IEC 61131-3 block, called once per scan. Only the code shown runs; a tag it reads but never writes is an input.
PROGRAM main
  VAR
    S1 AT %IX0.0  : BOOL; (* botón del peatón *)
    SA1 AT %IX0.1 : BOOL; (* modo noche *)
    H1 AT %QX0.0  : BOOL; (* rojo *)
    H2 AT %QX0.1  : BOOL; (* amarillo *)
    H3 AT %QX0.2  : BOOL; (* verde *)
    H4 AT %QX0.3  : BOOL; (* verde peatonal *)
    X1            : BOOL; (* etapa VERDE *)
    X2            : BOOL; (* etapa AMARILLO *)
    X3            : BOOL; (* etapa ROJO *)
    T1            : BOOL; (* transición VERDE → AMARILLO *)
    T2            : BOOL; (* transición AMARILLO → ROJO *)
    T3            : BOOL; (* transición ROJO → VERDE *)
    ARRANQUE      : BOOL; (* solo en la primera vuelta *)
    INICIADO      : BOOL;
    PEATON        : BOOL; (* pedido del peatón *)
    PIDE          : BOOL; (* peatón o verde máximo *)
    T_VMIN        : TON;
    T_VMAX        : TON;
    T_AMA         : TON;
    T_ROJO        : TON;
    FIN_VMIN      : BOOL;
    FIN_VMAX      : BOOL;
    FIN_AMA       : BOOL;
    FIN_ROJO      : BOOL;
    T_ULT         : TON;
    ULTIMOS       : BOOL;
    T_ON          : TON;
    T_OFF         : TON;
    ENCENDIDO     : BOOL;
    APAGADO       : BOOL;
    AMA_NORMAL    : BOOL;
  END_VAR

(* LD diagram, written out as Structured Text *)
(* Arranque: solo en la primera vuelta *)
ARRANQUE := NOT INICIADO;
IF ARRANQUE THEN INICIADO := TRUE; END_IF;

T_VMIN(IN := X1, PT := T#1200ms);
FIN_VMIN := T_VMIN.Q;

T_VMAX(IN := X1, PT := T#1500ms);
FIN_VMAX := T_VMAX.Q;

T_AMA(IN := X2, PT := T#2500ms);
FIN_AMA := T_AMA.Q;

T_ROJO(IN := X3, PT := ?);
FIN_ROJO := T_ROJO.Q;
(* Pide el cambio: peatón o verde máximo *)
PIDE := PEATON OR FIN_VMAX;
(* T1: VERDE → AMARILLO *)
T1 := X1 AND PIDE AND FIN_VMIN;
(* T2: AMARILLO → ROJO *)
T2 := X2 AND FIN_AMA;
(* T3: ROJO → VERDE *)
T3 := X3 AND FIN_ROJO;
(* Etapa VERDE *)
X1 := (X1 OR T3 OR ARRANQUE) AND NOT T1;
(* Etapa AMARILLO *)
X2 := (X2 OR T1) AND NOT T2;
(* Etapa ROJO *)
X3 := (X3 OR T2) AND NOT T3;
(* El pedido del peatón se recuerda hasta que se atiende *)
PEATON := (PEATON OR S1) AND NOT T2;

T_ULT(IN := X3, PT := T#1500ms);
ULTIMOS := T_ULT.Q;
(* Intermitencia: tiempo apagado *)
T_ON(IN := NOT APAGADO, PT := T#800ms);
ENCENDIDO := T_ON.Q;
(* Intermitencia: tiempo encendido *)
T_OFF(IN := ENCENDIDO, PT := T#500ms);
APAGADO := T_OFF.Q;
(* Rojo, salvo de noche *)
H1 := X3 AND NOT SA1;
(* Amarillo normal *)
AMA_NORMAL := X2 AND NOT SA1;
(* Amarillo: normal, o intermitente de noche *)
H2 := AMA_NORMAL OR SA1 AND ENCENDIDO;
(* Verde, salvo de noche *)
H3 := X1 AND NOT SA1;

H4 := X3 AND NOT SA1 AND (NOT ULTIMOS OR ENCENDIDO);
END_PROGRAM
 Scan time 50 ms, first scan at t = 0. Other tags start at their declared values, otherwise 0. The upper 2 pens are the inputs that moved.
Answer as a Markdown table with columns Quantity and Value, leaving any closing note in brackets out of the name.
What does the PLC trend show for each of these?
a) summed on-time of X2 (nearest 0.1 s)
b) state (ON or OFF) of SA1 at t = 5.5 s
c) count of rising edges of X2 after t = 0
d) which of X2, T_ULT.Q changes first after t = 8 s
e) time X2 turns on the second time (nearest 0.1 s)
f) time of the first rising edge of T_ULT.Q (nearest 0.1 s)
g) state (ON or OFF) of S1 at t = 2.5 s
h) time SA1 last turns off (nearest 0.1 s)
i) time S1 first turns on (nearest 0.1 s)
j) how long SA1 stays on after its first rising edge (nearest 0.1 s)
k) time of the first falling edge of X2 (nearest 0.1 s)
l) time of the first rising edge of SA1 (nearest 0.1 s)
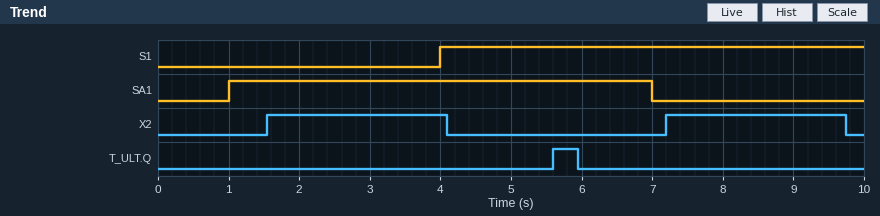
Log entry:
| Quantity | Value |
|---|---|
| summed on-time of X2 | 5.1 s |
| state (ON or OFF) of SA1 at t = 5.5 s | ON |
| count of rising edges of X2 after t = 0 | 2 |
| which of X2, T_ULT.Q changes first after t = 8 s | X2 |
| time X2 turns on the second time | 7.2 s |
| time of the first rising edge of T_ULT.Q | 5.6 s |
| state (ON or OFF) of S1 at t = 2.5 s | OFF |
| time SA1 last turns off | 7.0 s |
| time S1 first turns on | 4.0 s |
| how long SA1 stays on after its first rising edge | 6.0 s |
| time of the first falling edge of X2 | 4.1 s |
| time of the first rising edge of SA1 | 1.0 s |
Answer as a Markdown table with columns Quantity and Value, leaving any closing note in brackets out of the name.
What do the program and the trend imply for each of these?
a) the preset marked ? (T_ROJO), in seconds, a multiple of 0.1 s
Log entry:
| Quantity | Value |
|---|---|
| the preset marked ? (T_ROJO), in seconds, a multiple of 0.1 s | 1.8 s |
